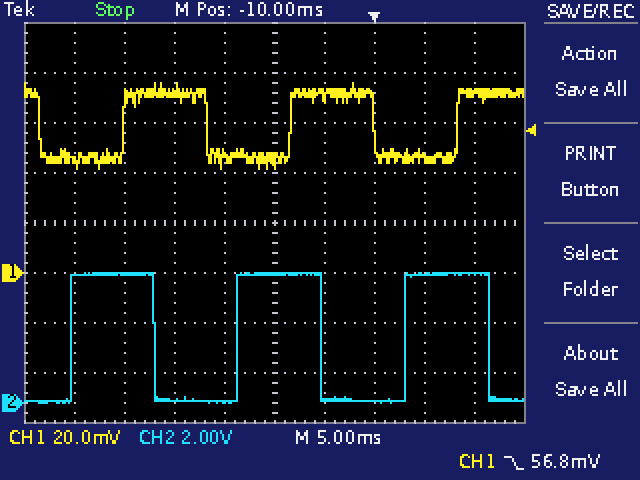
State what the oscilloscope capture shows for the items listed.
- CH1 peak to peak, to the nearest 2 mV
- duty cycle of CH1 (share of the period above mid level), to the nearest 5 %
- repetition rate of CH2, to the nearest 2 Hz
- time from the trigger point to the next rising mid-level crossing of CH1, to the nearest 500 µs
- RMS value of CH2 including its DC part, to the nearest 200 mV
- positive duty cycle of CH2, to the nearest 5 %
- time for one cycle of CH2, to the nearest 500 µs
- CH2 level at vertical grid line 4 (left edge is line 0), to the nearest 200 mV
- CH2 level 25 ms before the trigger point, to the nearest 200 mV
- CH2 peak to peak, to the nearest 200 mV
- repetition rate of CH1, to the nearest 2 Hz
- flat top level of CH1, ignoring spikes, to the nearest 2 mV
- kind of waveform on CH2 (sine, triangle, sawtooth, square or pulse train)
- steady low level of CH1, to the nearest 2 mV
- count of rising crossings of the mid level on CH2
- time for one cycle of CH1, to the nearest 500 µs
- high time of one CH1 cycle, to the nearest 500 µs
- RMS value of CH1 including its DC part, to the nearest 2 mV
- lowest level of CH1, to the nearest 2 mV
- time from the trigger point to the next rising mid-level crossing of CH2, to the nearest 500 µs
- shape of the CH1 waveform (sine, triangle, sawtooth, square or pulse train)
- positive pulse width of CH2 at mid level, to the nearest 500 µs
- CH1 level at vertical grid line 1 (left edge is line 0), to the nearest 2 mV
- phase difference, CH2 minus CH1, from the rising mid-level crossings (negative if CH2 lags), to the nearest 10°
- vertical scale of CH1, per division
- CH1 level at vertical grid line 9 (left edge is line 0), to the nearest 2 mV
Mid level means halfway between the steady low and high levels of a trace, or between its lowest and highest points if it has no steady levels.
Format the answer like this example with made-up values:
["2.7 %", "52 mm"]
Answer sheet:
["34 mV", "50 %", "60 Hz", "8.5 ms", "3.6 V", "50 %", "16.5 ms", "0.0 V", "5.2 V", "5.2 V", "60 Hz", "72 mV", "square", "46 mV", "3", "16.5 ms", "8.5 ms", "60 mV", "42 mV", "3.0 ms", "square", "8.5 ms", "44 mV", "+110°", "20 mV", "72 mV"]
